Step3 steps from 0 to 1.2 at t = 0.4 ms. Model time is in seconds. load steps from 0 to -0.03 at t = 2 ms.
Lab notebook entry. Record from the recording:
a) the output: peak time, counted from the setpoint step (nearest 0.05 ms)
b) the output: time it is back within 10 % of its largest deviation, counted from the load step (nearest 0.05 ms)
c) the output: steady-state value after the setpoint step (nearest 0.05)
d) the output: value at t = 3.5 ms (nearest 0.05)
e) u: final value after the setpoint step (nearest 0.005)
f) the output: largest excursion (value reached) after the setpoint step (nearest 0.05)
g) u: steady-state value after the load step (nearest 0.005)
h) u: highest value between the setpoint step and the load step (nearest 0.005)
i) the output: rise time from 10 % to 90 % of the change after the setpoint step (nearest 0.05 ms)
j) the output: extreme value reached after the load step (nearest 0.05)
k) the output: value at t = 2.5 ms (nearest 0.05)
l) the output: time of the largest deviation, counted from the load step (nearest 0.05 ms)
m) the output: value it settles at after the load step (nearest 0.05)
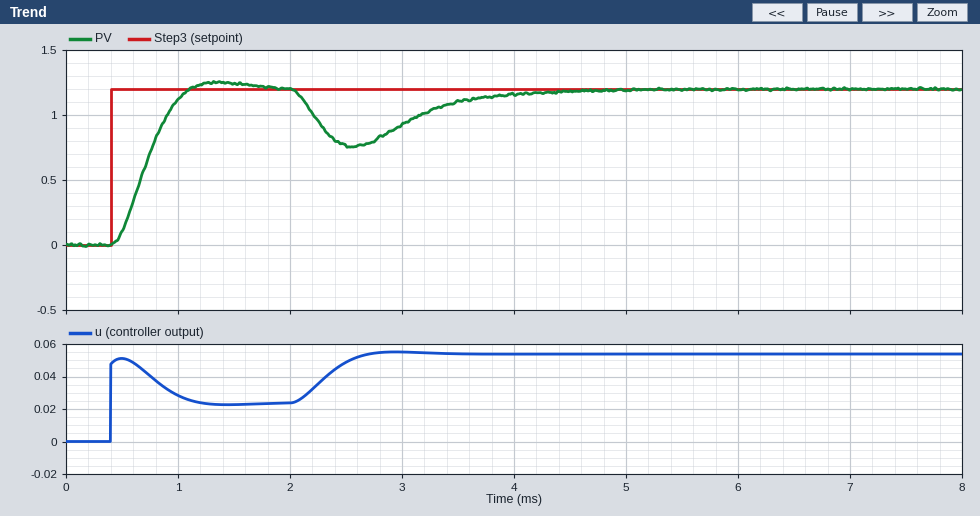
0.95 ms
1.95 ms
1.20
1.10
0.025
1.25
0.055
0.050
0.45 ms
0.75
0.75
0.55 ms
1.20
